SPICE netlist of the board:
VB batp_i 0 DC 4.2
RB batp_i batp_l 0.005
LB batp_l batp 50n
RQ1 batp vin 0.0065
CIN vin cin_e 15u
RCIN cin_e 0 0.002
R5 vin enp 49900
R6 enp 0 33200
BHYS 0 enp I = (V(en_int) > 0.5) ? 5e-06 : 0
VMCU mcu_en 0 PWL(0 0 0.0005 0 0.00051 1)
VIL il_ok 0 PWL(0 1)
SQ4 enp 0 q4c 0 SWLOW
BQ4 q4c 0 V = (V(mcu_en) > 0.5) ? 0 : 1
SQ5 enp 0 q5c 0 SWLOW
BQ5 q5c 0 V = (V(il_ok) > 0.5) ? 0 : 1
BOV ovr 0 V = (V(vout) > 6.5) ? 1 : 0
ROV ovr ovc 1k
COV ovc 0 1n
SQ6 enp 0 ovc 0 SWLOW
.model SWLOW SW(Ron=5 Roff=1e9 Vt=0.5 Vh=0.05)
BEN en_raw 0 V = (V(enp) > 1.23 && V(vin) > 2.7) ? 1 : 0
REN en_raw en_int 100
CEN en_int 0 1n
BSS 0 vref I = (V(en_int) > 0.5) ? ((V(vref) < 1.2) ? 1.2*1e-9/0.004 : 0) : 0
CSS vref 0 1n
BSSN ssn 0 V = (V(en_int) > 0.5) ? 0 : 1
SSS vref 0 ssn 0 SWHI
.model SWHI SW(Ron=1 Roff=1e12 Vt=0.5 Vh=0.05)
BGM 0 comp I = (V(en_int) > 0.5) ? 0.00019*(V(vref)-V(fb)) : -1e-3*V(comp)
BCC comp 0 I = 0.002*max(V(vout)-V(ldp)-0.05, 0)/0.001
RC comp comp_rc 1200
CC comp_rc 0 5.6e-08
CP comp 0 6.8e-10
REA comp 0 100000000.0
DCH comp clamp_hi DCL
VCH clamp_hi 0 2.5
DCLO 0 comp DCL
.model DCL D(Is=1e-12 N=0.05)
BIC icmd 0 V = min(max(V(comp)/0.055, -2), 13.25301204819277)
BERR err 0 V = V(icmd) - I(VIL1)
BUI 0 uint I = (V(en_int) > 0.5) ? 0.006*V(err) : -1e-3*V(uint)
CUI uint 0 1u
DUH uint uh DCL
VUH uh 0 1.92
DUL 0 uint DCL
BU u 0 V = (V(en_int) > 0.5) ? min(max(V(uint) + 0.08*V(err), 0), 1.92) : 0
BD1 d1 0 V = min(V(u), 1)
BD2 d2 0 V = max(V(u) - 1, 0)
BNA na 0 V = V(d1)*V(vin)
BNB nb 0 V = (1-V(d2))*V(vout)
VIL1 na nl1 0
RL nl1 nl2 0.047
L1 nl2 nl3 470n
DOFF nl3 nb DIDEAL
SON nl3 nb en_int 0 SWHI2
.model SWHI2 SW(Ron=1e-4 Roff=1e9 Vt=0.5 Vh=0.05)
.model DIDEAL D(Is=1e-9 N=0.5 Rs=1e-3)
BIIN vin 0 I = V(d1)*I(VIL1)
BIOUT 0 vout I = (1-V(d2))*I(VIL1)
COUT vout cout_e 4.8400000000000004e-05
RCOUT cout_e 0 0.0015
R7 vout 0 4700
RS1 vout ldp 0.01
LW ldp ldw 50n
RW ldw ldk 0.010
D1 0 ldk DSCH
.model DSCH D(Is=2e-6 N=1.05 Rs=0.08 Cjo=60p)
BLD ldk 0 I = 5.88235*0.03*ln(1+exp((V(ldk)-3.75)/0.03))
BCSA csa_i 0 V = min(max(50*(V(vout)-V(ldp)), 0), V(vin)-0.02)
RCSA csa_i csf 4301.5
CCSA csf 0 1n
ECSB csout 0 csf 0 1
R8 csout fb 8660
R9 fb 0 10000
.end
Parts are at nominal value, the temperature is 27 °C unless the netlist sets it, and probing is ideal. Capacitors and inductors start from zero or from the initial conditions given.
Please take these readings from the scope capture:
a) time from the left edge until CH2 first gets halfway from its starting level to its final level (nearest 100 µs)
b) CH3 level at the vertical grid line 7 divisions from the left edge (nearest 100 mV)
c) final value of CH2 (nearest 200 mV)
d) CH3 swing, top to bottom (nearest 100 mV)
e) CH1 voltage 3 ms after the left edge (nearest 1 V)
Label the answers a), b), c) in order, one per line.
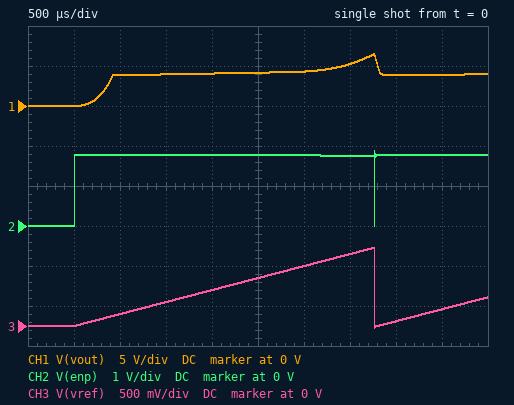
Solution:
a) 500 µs
b) 900 mV
c) 1.8 V
d) 1.0 V
e) 4 V
